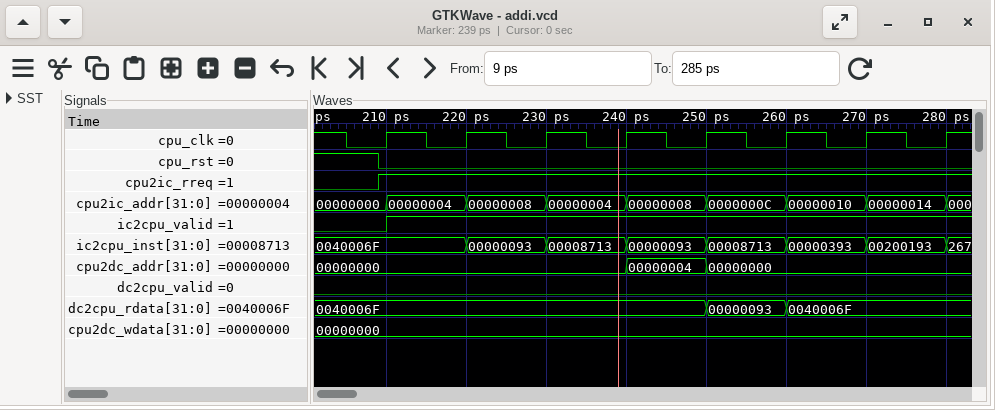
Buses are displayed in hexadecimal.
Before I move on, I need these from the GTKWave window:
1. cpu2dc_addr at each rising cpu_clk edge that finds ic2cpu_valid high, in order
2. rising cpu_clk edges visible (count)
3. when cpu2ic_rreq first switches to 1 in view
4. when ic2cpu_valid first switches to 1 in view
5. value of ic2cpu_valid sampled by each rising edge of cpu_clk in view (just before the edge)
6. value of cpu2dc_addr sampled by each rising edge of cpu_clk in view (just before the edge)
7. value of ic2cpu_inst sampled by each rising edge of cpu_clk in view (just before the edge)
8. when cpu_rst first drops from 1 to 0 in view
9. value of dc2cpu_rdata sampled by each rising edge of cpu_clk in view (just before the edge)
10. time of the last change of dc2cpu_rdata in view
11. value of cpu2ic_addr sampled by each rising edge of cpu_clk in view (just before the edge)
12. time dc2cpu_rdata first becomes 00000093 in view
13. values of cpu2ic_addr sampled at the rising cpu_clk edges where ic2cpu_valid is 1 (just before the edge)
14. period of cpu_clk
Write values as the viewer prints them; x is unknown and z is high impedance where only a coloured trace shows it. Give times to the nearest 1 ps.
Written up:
00000000, 00000000, 00000000, 00000004, 00000000, 00000000, 00000000
8
209 ps
210 ps
0 1 1 1 1 1 1 1
00000000, 00000000, 00000000, 00000000, 00000004, 00000000, 00000000, 00000000
0040006F, 0040006F, 00000093, 00008713, 00000093, 00008713, 00000393, 00200193
209 ps
0040006F, 0040006F, 0040006F, 0040006F, 0040006F, 00000093, 0040006F, 0040006F
260 ps
00000000, 00000004, 00000008, 00000004, 00000008, 0000000C, 00000010, 00000014
250 ps
00000004, 00000008, 00000004, 00000008, 0000000C, 00000010, 00000014
10 ps
